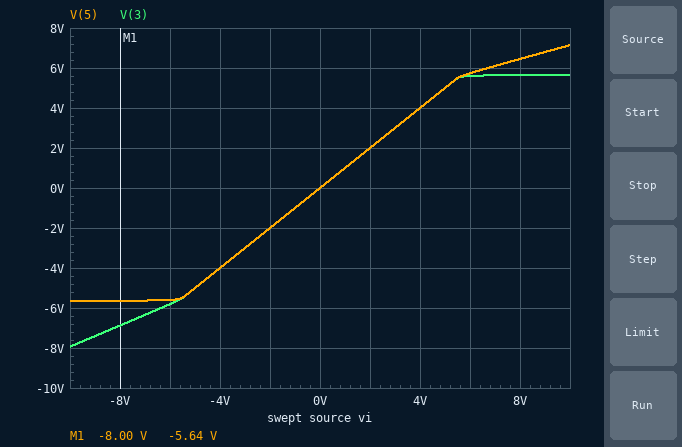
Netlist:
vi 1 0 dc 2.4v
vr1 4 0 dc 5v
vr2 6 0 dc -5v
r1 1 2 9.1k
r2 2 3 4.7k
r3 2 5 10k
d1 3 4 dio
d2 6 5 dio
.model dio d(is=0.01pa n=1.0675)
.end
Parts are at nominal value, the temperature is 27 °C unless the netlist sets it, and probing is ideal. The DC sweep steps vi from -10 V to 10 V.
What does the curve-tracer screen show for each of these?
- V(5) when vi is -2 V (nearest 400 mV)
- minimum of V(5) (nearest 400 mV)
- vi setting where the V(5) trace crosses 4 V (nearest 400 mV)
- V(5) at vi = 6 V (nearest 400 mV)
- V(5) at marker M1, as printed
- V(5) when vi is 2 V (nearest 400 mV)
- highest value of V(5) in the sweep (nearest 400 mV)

-2.0 V
-5.6 V
4.0 V
5.6 V
-5.64 V
2.0 V
7.2 V
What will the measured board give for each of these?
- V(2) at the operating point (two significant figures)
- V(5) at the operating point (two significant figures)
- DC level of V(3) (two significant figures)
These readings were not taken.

2.4 V
2.4 V
2.4 V
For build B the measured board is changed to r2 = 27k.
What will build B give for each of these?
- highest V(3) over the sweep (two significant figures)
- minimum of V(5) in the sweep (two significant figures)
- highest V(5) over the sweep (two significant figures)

5.6 V
-5.7 V
8.9 V
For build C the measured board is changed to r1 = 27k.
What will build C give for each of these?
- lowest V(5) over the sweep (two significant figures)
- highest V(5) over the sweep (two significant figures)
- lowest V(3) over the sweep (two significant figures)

-5.6 V
6.3 V
-6.8 V
